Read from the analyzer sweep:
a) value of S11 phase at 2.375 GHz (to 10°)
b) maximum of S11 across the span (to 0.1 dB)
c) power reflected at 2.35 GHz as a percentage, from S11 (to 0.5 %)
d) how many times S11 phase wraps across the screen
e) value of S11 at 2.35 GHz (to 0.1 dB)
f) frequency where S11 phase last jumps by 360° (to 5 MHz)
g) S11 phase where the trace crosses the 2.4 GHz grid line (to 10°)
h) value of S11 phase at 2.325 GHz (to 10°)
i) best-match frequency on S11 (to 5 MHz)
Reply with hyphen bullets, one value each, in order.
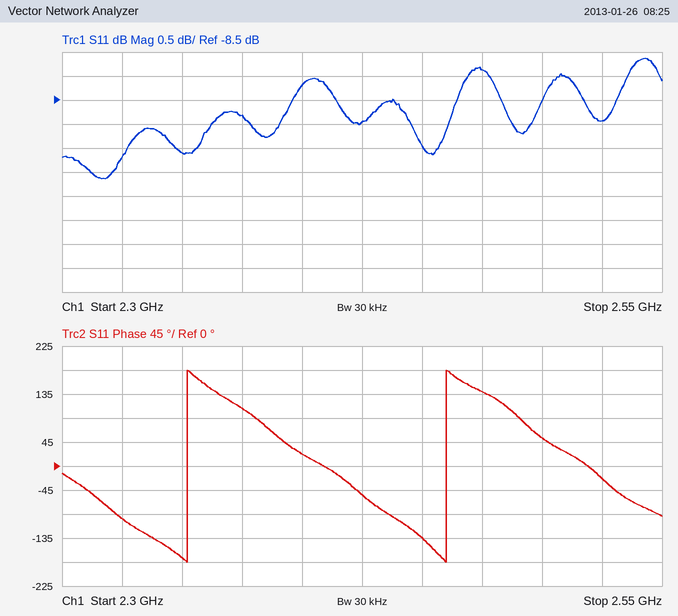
- 110°
- -7.6 dB
- 11.0 %
- 2
- -9.6 dB
- 2.460 GHz
- 20°
- -100°
- 2.315 GHz
